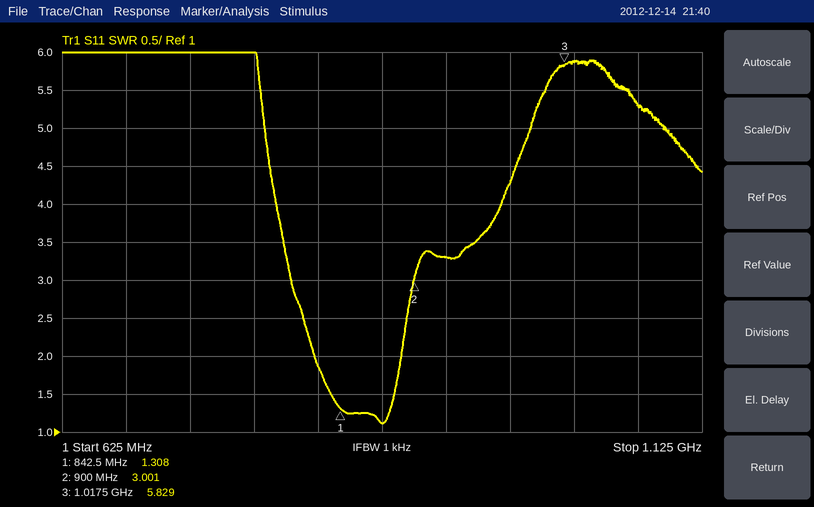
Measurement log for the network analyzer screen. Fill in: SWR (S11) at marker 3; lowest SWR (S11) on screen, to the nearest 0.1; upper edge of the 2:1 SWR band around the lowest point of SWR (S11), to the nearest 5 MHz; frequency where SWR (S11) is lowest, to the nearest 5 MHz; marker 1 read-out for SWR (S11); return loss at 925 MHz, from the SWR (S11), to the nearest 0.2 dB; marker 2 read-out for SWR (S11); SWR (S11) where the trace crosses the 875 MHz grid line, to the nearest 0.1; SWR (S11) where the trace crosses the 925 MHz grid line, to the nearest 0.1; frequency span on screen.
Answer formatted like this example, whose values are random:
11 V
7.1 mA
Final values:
5.829
1.1
890 MHz
875 MHz
1.308
5.4 dB
3.001
1.1
3.3
500 MHz
